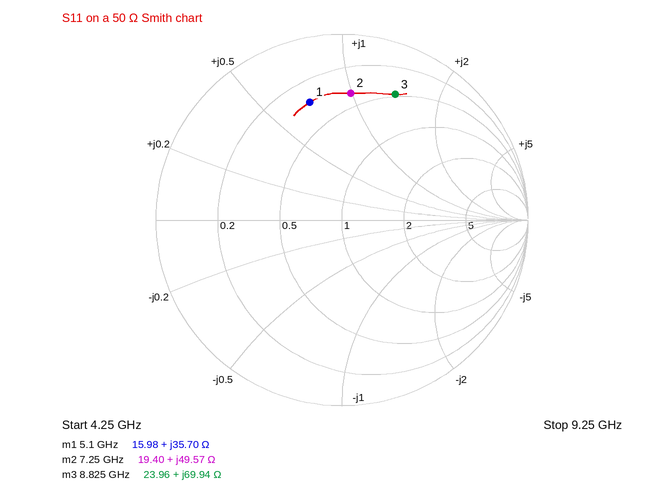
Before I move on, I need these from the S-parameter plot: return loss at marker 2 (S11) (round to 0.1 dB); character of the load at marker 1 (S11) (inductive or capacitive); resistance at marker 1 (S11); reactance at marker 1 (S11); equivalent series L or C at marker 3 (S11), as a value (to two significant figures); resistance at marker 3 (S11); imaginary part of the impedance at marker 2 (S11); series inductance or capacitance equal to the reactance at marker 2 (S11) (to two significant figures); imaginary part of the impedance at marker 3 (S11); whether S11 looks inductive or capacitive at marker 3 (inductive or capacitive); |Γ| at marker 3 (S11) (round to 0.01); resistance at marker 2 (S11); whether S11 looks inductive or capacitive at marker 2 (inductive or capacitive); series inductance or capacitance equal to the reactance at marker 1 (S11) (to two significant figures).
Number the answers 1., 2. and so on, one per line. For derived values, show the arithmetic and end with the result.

1. 3.3 dB
2. inductive
3. 15.98 Ω
4. +35.70 Ω
5. L = 69.94 Ω/(2π × 8.825 GHz) ≈ 1.3 nH
6. 23.96 Ω
7. +49.57 Ω
8. L = 49.57 Ω/(2π × 7.25 GHz) ≈ 1.1 nH
9. +69.94 Ω
10. inductive
11. 0.73
12. 19.40 Ω
13. inductive
14. L = 35.7 Ω/(2π × 5.1 GHz) ≈ 1.1 nH
